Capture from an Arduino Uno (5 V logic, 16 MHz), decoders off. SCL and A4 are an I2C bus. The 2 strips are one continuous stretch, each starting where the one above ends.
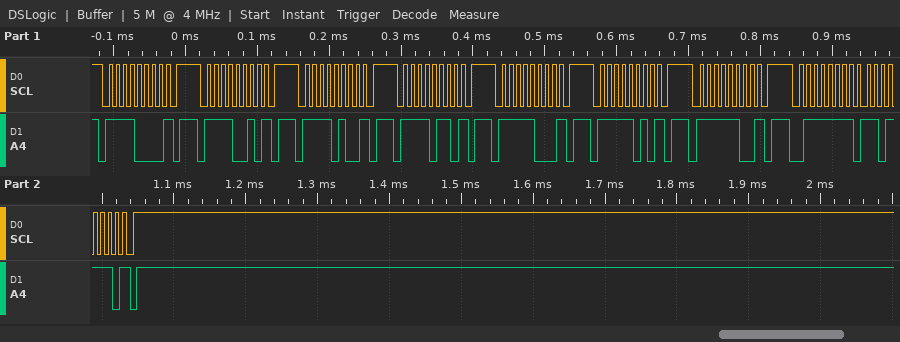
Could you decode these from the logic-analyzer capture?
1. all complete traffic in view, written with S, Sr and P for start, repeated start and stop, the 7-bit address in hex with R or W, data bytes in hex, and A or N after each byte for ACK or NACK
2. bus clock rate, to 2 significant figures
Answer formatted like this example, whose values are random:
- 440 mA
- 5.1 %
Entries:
- S 78W N P S 79W N P S 7AW N P S 7BW N P S 7CW N P S 7DW N P S 7EW N P S 3FR A DE N P
- 100 kHz
